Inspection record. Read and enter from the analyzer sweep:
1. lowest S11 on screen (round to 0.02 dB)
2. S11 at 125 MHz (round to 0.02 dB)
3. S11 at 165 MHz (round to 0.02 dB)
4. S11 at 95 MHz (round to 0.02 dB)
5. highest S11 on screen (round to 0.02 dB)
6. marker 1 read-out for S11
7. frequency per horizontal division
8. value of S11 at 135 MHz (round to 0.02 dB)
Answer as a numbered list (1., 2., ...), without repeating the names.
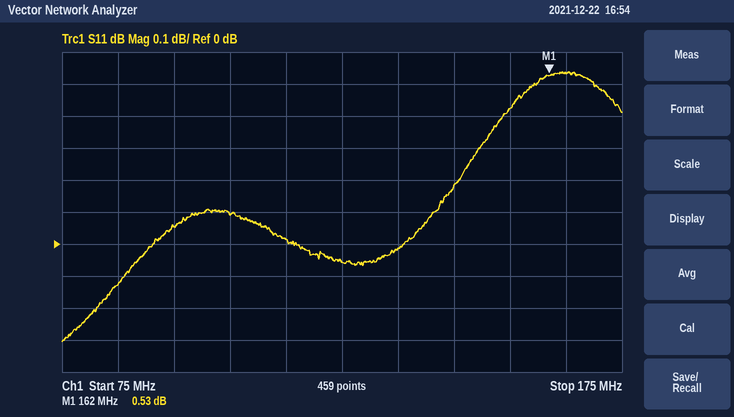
1. -0.30 dB
2. -0.06 dB
3. 0.54 dB
4. 0.06 dB
5. 0.54 dB
6. 0.53 dB
7. 10 MHz
8. -0.02 dB
